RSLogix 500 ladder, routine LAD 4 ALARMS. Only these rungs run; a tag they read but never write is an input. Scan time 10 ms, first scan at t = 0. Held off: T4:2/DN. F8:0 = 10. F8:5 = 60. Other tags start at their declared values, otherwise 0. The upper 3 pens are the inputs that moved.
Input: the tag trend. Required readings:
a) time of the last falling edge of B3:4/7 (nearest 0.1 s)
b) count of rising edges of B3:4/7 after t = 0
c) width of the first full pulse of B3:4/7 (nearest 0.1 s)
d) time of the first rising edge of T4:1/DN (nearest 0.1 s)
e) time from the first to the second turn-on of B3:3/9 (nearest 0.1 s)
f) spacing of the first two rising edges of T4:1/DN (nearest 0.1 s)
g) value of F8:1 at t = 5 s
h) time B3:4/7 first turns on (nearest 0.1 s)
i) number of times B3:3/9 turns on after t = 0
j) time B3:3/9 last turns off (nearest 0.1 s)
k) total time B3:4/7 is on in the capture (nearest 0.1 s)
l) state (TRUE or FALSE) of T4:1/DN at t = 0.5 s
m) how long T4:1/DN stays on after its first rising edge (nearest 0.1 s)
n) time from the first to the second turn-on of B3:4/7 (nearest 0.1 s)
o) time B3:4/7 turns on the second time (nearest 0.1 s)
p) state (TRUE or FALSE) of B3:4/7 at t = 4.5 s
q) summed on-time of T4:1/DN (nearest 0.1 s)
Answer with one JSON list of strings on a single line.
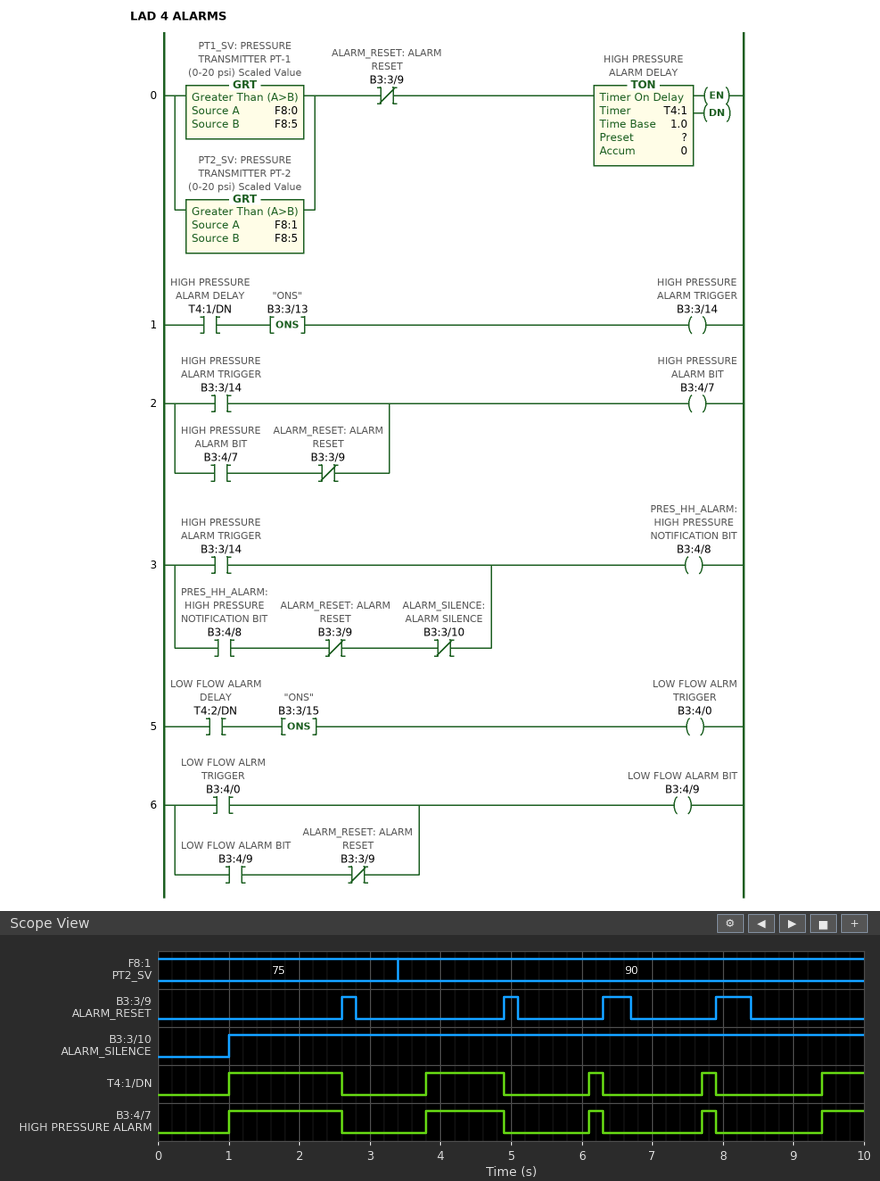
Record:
["7.9 s", "5", "1.6 s", "1.0 s", "2.3 s", "2.8 s", "90", "1.0 s", "4", "8.4 s", "3.7 s", "FALSE", "1.6 s", "2.8 s", "3.8 s", "TRUE", "3.7 s"]
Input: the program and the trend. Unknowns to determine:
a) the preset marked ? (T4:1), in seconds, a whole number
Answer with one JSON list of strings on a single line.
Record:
["1 s"]
